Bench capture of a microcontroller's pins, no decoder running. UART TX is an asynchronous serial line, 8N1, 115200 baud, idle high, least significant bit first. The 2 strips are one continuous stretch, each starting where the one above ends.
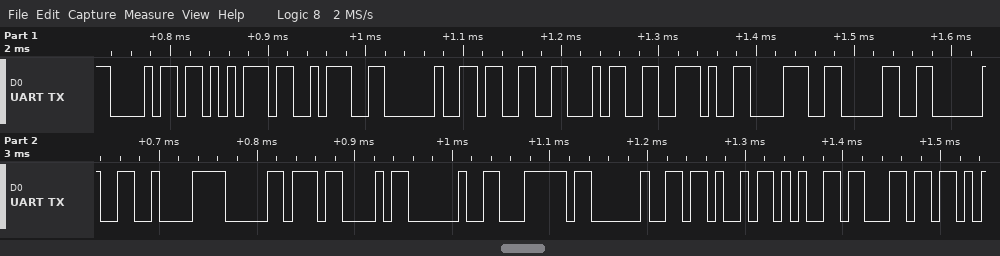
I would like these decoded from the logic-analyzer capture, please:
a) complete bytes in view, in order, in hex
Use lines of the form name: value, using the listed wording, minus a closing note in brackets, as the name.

complete bytes in view, in order, in hex: 0x68 0x75 0x3A 0x20 0x33 0x34 0x2E 0x38 0x30 0x20 0xC2 0xB0 0x43 0x20 0x7C 0x20 0x4B 0x65 0x6C
